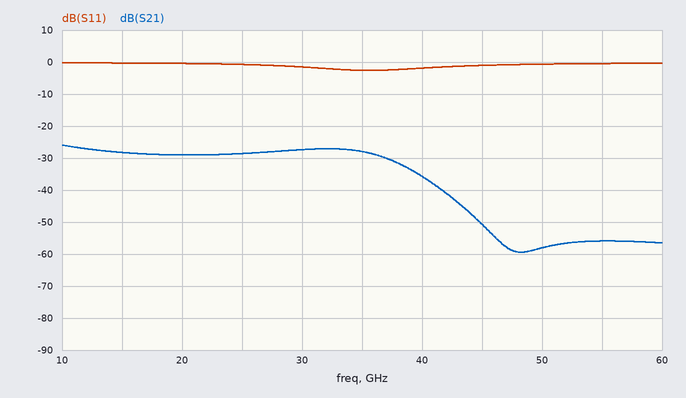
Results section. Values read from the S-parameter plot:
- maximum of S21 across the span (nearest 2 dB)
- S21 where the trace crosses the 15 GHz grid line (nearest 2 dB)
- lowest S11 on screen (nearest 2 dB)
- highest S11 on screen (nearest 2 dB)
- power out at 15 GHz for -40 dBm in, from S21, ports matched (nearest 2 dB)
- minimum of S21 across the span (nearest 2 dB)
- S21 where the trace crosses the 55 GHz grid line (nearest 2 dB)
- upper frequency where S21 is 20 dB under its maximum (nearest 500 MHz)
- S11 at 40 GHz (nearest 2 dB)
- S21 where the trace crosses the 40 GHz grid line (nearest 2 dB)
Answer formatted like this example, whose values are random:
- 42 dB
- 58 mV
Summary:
- -26 dB
- -28 dB
- -2 dB
- 0 dB
- -68 dBm
- -60 dB
- -56 dB
- 43.5 GHz
- -2 dB
- -36 dB
